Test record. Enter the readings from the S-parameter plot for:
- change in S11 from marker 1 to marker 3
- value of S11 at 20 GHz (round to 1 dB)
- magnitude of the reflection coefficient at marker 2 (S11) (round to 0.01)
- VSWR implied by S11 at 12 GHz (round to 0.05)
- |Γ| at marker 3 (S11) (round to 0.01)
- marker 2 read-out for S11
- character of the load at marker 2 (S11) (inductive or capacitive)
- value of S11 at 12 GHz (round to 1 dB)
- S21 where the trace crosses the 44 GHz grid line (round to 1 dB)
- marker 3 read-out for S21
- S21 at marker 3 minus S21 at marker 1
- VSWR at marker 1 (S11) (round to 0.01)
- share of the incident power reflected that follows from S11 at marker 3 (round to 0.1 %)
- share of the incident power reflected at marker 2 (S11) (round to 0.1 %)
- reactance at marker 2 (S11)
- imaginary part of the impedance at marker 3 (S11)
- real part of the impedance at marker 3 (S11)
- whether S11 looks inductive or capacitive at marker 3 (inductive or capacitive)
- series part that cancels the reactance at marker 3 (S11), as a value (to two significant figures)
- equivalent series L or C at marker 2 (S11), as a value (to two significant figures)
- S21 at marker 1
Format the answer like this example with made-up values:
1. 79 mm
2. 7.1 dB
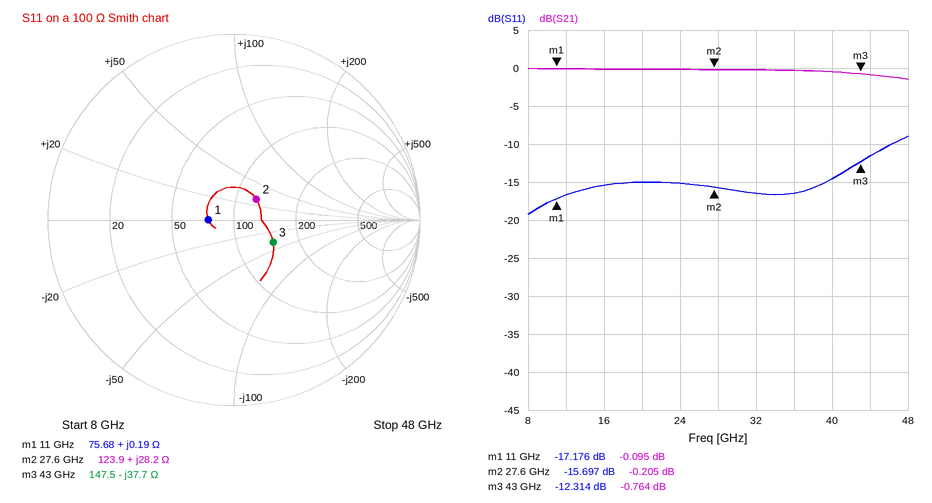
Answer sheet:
1. 4.862 dB
2. -15 dB
3. 0.16
4. 1.35
5. 0.24
6. -15.697 dB
7. inductive
8. -17 dB
9. -1 dB
10. -0.764 dB
11. -0.669 dB
12. 1.32
13. 5.9 %
14. 2.7 %
15. +28.2 Ω
16. -37.7 Ω
17. 147.5 Ω
18. capacitive
19. 140 pH
20. 160 pH
21. -0.095 dB
